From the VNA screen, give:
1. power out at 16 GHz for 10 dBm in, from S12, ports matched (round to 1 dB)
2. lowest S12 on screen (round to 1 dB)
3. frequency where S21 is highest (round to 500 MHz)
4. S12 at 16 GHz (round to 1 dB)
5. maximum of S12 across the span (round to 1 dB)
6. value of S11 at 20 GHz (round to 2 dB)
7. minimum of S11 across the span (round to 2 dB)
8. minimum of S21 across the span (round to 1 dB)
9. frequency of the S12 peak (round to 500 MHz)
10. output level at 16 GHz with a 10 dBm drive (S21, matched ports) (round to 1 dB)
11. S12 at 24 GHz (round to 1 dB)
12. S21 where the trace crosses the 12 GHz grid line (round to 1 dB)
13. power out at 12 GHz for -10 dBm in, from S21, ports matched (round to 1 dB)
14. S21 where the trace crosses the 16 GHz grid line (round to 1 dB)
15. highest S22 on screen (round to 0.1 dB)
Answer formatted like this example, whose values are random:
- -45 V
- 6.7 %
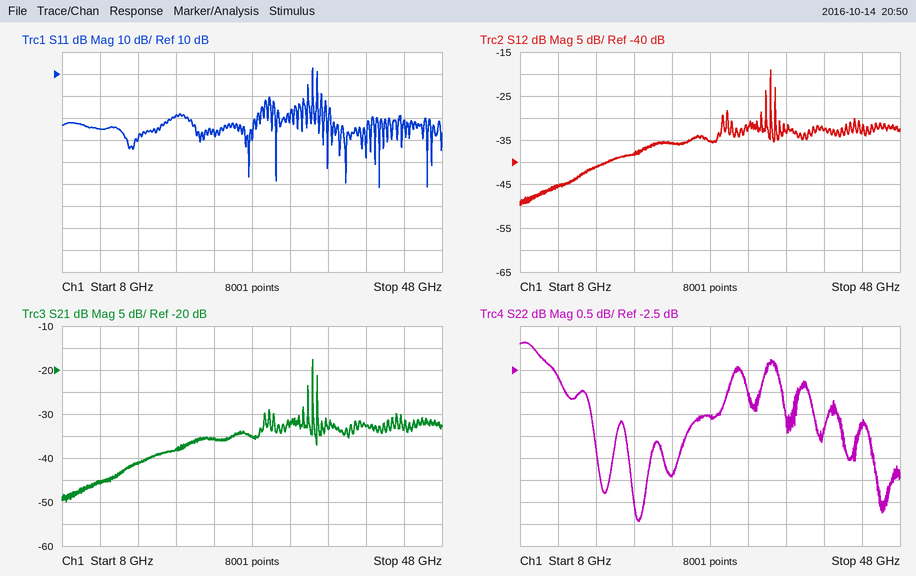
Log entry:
- -31 dBm
- -50 dB
- 34.5 GHz
- -41 dB
- -19 dB
- -8 dB
- -42 dB
- -50 dB
- 34.5 GHz
- -31 dBm
- -36 dB
- -45 dB
- -55 dBm
- -41 dB
- -1.9 dB
